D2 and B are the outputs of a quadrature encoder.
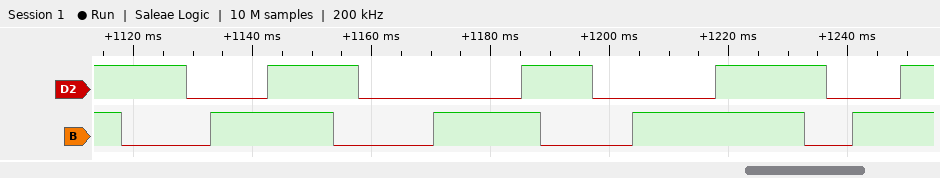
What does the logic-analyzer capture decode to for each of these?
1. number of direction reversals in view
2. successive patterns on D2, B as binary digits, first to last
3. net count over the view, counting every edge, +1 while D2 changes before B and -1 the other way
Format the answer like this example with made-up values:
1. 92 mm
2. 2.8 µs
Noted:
1. 0
2. 11 10 00 01 11 10 00 01 11 10 00 01 11 10 00 01 11
3. -16
